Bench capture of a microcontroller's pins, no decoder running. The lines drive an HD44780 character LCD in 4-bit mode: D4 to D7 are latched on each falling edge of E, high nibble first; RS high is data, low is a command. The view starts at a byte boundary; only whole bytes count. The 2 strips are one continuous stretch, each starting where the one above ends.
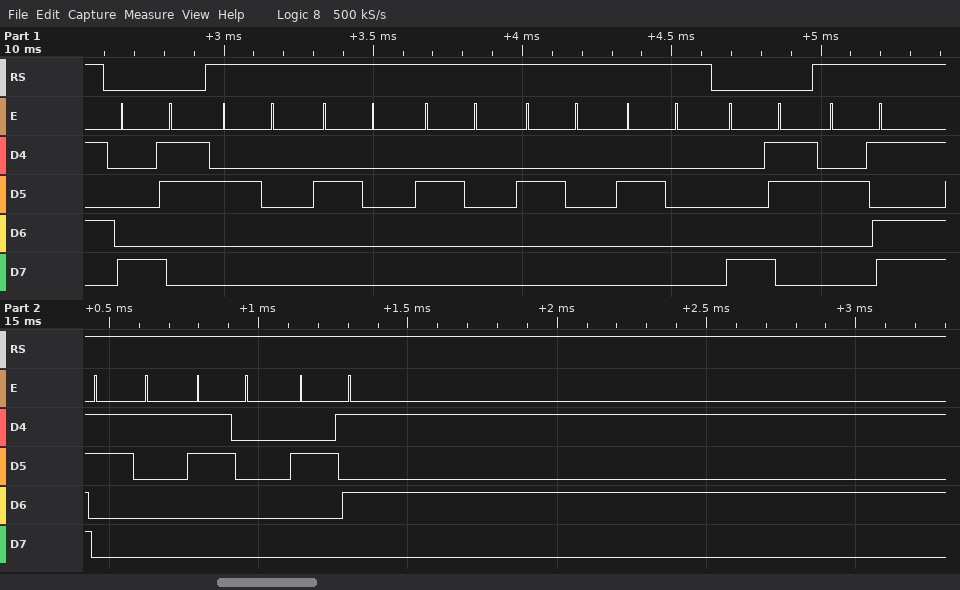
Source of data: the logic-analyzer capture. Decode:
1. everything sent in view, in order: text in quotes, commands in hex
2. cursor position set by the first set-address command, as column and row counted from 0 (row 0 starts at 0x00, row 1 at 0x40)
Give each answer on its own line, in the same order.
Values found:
0x83 "     " 0x83 "-10%"
column 3, row 0
